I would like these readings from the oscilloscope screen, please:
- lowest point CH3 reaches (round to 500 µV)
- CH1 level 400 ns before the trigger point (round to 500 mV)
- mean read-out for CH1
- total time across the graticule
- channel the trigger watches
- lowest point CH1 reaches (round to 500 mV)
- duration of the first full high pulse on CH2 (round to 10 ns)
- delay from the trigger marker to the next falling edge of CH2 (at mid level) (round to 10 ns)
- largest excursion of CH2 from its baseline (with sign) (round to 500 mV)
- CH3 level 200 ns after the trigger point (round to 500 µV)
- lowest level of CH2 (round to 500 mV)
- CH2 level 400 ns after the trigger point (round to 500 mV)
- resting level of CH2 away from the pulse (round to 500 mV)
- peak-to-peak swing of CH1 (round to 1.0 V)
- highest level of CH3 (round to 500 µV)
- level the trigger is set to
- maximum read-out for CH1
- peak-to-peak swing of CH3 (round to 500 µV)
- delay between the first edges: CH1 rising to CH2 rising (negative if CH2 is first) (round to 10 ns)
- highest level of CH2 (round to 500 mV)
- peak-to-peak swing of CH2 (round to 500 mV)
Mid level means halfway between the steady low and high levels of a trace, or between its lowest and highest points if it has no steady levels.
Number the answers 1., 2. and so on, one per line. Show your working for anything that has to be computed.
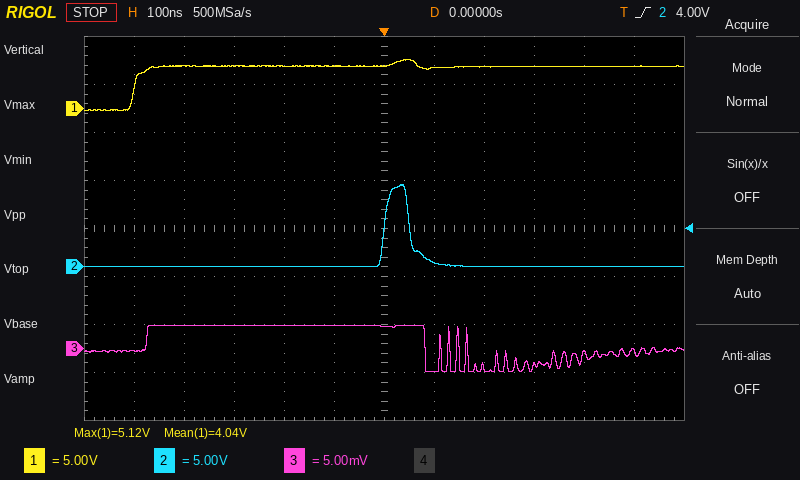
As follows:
1. -2.5 mV
2. 4.5 V
3. 4.04 V
4. 1.2 µs
5. CH2
6. 0.0 V
7. 50 ns
8. 50 ns
9. 8.5 V − (0.0 V) = +8.5 V
10. -2.0 mV
11. 0.0 V
12. 0.0 V
13. 0.0 V
14. 5.0 V
15. 2.5 mV
16. 4.00 V
17. 5.12 V
18. 2.5 mV − (-2.5 mV) = 5.0 mV
19. +500 ns
20. 8.5 V
21. 8.5 V − (0.0 V) = 8.5 V
